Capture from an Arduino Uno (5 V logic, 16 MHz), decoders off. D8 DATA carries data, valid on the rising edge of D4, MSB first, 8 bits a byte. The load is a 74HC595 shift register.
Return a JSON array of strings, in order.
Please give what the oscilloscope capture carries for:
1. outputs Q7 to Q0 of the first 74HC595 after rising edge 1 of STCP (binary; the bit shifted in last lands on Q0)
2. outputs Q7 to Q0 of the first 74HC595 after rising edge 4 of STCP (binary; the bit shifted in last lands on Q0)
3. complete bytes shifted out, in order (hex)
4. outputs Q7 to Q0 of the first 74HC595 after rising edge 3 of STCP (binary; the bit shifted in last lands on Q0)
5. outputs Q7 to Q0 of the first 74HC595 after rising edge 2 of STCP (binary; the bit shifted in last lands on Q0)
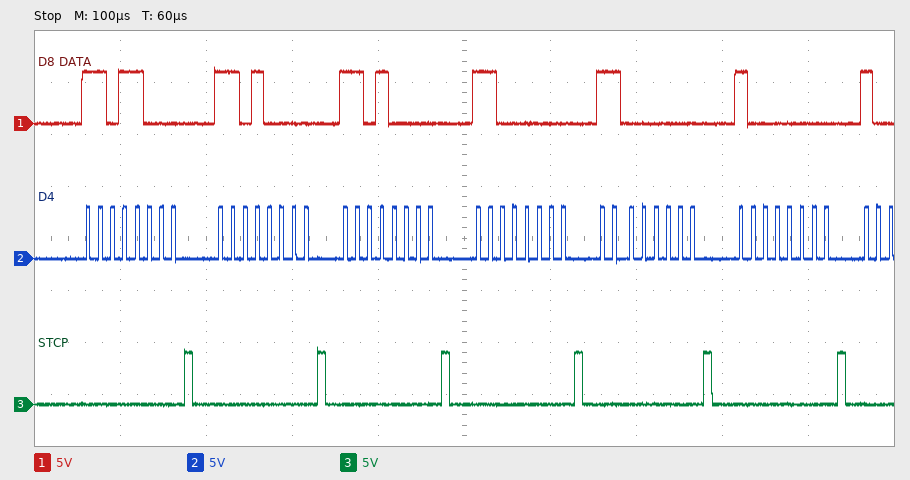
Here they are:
["11011000", "11000000", "D8 D0 D0 C0 C0 80", "11010000", "11010000"]
